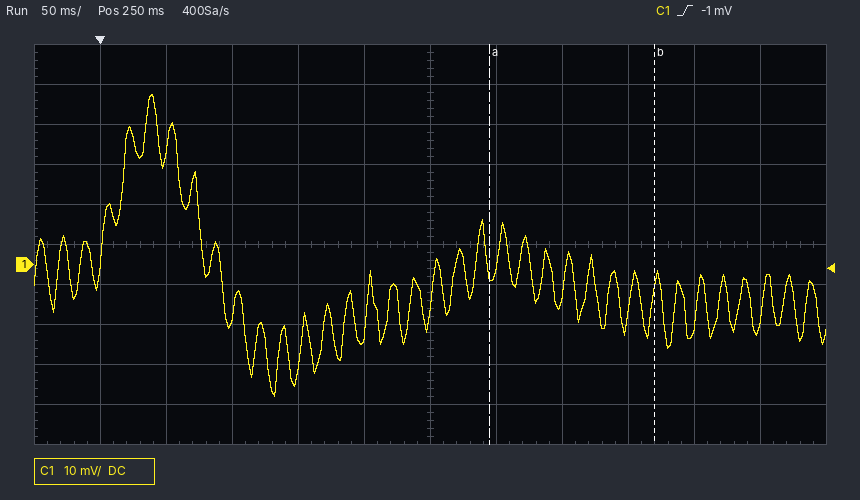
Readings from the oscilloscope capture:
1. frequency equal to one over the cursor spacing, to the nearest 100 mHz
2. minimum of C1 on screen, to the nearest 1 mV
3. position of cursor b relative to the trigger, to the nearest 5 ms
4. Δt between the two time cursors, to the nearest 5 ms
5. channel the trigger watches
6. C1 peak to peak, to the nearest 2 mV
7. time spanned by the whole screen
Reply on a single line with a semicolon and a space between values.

8.0 Hz; -33 mV; +420 ms; 125 ms; C1; 76 mV; 600 ms
